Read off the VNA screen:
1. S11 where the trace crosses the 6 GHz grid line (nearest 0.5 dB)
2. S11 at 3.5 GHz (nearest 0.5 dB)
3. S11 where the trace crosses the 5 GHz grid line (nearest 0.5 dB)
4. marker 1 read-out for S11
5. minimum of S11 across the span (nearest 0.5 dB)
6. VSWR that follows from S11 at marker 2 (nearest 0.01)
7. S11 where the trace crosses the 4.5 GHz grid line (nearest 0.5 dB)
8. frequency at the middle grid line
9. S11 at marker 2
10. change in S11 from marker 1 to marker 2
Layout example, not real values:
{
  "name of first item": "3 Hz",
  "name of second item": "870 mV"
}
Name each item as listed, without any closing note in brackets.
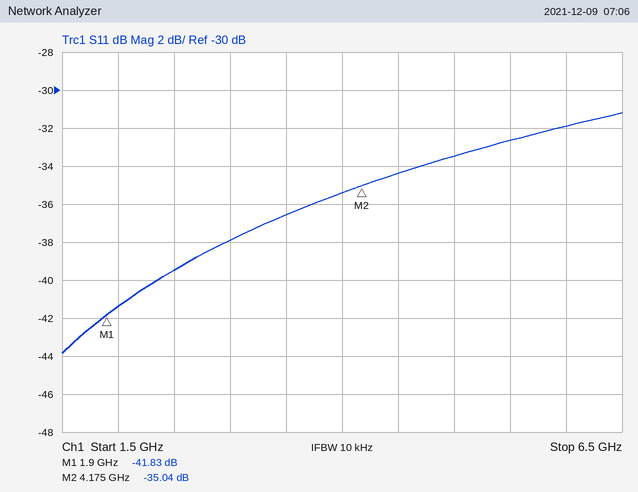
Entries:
{
  "S11 where the trace crosses the 6 GHz grid line": "-32.0 dB",
  "S11 at 3.5 GHz": "-36.5 dB",
  "S11 where the trace crosses the 5 GHz grid line": "-33.5 dB",
  "marker 1 read-out for S11": "-41.83 dB",
  "minimum of S11 across the span": "-44.0 dB",
  "VSWR that follows from S11 at marker 2": "1.04",
  "S11 where the trace crosses the 4.5 GHz grid line": "-34.5 dB",
  "frequency at the middle grid line": "4 GHz",
  "S11 at marker 2": "-35.04 dB",
  "change in S11 from marker 1 to marker 2": "6.79 dB"
}
